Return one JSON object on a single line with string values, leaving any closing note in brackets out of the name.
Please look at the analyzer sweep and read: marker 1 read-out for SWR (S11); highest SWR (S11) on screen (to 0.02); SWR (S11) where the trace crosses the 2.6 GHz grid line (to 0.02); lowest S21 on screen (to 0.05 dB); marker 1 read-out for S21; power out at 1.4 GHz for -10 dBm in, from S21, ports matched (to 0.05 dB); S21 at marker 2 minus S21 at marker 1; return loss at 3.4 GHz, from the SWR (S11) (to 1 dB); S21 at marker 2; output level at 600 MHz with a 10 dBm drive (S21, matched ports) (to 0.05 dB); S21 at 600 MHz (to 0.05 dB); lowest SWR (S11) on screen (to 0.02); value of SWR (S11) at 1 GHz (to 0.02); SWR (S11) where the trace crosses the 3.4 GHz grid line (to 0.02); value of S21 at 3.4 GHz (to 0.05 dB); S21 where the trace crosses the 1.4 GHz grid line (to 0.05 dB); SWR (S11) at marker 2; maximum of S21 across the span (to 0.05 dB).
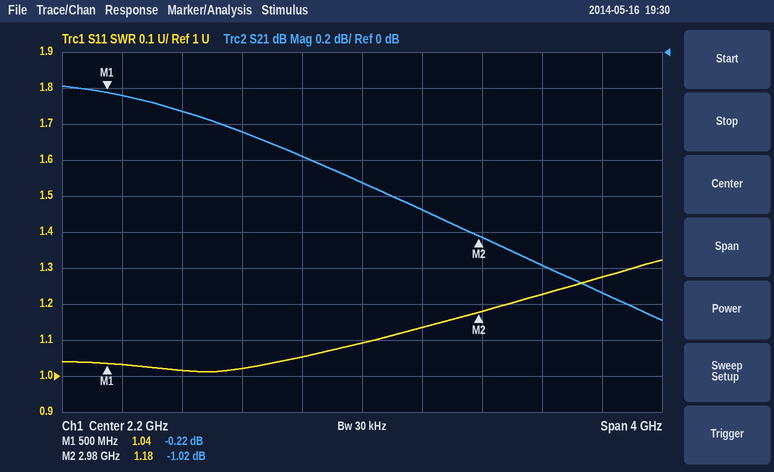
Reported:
{"marker 1 read-out for SWR": "1.04", "highest SWR (S11) on screen": "1.32", "SWR (S11) where the trace crosses the 2.6 GHz grid line": "1.14", "lowest S21 on screen": "-1.50 dB", "marker 1 read-out for S21": "-0.22 dB", "power out at 1.4 GHz for -10 dBm in, from S21, ports matched": "-10.45 dBm", "S21 at marker 2 minus S21 at marker 1": "-0.80 dB", "return loss at 3.4 GHz, from the SWR (S11)": "20 dB", "S21 at marker 2": "-1.02 dB", "output level at 600 MHz with a 10 dBm drive (S21, matched ports)": "9.75 dBm", "S21 at 600 MHz": "-0.25 dB", "lowest SWR (S11) on screen": "1.02", "value of SWR (S11) at 1 GHz": "1.02", "SWR (S11) where the trace crosses the 3.4 GHz grid line": "1.22", "value of S21 at 3.4 GHz": "-1.20 dB", "S21 where the trace crosses the 1.4 GHz grid line": "-0.45 dB", "SWR (S11) at marker 2": "1.18", "maximum of S21 across the span": "-0.20 dB"}
